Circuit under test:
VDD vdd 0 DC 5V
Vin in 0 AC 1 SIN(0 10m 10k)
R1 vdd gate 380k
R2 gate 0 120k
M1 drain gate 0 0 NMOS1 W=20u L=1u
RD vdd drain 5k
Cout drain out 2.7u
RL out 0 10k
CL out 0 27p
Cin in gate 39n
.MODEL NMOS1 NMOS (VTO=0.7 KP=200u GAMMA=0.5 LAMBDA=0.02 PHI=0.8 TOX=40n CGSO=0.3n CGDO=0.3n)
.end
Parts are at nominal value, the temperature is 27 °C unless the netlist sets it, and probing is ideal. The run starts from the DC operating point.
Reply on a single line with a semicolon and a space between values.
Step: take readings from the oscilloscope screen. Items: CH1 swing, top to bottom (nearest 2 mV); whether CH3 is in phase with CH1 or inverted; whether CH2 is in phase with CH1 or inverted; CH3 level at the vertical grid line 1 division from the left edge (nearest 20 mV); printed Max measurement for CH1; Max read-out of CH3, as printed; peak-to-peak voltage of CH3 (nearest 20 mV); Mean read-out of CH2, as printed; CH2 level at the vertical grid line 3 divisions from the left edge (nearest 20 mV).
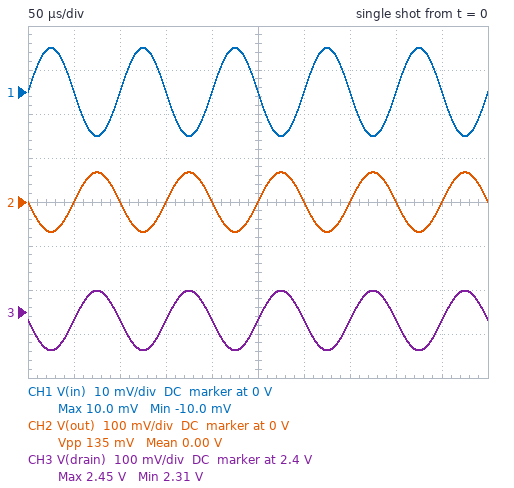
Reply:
20 mV; inverted; inverted; 2.38 V; 10.0 mV; 2.45 V; 140 mV; 0.00 V; 0 V
